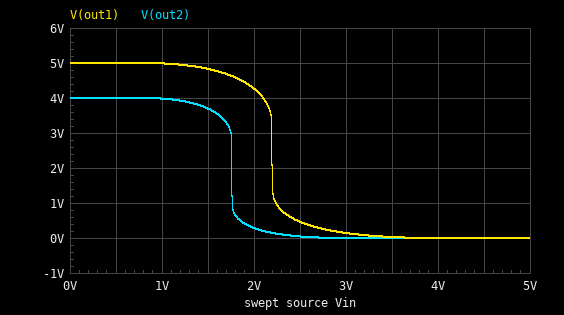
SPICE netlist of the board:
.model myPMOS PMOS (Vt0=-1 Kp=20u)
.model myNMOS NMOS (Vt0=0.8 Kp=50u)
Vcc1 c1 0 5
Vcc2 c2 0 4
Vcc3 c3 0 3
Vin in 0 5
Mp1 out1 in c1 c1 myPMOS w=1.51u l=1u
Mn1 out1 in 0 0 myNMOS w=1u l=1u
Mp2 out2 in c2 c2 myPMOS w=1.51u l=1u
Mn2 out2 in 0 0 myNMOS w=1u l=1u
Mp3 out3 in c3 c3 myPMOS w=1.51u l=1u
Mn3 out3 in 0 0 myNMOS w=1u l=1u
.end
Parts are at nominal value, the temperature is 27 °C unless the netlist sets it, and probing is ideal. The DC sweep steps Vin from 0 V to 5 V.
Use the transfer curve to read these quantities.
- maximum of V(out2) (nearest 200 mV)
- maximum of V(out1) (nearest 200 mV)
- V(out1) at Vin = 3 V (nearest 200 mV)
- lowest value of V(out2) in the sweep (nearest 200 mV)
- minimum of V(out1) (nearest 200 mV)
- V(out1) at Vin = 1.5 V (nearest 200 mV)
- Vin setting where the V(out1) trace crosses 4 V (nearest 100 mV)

4.0 V
5.0 V
200 mV
0 V
0 V
4.8 V
2.1 V
